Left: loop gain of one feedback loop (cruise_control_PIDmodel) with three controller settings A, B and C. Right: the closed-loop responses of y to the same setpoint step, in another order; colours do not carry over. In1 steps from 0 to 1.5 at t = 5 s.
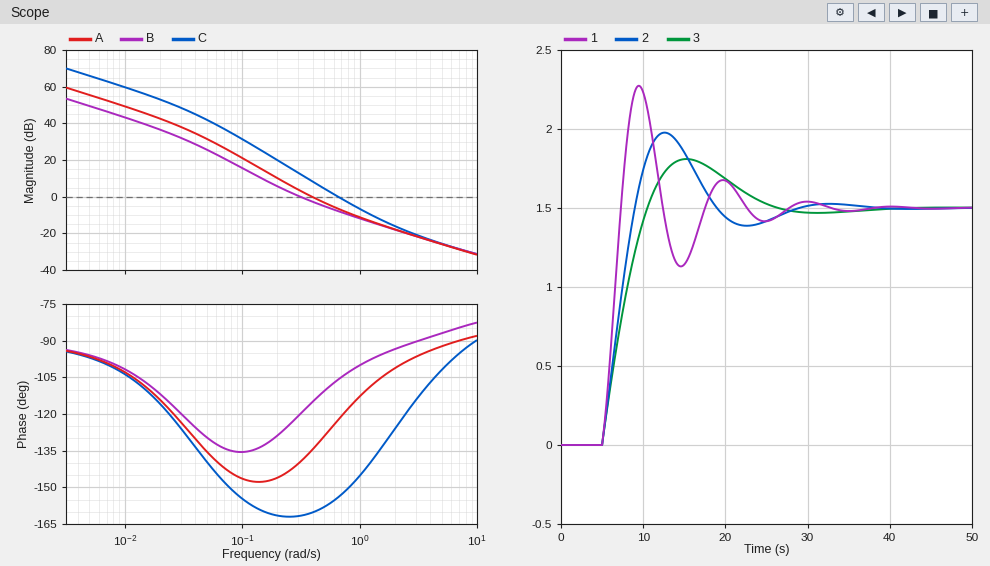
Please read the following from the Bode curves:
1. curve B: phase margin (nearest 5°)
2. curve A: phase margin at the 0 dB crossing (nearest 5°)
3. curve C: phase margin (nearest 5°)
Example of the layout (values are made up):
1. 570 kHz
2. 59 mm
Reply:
1. 60°
2. 45°
3. 25°
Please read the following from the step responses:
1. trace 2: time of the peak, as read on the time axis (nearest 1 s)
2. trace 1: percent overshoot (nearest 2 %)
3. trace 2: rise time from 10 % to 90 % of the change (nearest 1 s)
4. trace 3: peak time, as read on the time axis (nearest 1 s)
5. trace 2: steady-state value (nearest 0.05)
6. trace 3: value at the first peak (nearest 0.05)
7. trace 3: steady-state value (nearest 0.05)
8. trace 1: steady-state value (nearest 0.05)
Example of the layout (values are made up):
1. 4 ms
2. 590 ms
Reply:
1. 13 s
2. 52 %
3. 3 s
4. 15 s
5. 1.50
6. 1.80
7. 1.50
8. 1.50
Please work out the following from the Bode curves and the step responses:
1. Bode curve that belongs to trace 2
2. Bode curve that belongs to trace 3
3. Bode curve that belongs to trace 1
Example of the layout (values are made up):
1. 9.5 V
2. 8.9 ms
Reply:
1. A
2. B
3. C
